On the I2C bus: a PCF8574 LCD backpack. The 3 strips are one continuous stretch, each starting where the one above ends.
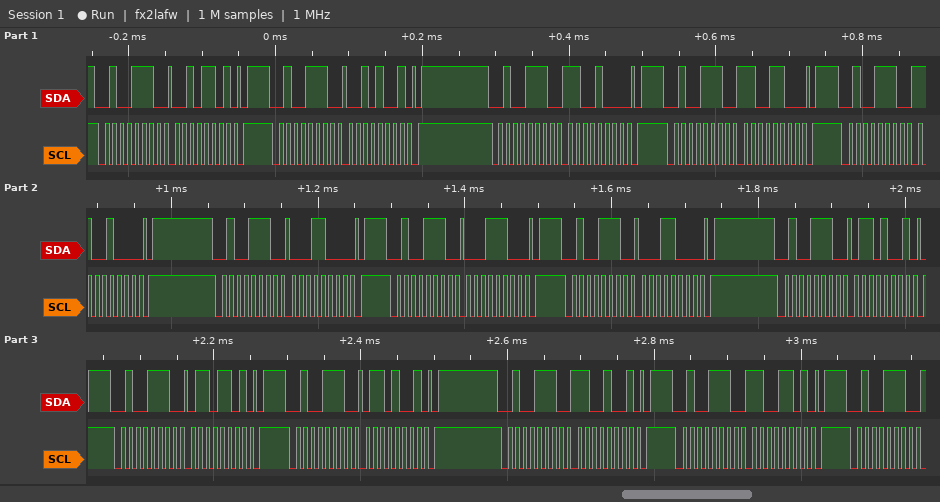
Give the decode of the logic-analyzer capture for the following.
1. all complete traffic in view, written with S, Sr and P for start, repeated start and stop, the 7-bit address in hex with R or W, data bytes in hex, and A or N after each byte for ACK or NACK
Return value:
S 27W A 2D A P S 27W A 29 A P S 27W A C8 A P S 27W A CC A P S 27W A C8 A P S 27W A 18 A P S 27W A 1C A P S 27W A 18 A P S 27W A 69 A P S 27W A 6D A P S 27W A 69 A P S 27W A C9 A P S 27W A CD A P S 27W A
